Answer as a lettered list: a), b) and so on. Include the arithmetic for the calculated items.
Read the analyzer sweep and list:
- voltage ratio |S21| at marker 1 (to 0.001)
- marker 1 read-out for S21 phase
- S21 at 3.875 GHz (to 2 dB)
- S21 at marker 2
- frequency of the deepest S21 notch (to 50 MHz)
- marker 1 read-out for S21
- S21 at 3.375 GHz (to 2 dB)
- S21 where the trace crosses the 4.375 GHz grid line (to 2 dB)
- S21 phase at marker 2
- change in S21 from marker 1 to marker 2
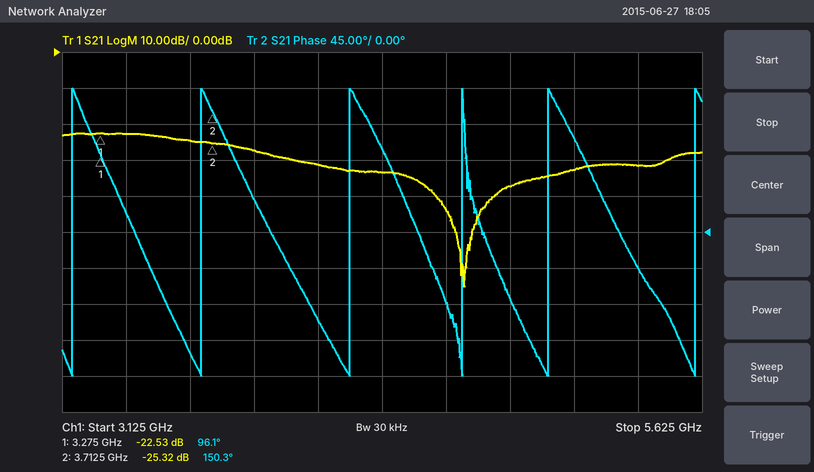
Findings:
a) 10^(-22.53/20) ≈ 0.075
b) 96.1°
c) -28 dB
d) -25.32 dB
e) 4.70 GHz
f) -22.53 dB
g) -22 dB
h) -34 dB
i) 150.3°
j) -25.32 − (-22.53) = -2.79 dB
